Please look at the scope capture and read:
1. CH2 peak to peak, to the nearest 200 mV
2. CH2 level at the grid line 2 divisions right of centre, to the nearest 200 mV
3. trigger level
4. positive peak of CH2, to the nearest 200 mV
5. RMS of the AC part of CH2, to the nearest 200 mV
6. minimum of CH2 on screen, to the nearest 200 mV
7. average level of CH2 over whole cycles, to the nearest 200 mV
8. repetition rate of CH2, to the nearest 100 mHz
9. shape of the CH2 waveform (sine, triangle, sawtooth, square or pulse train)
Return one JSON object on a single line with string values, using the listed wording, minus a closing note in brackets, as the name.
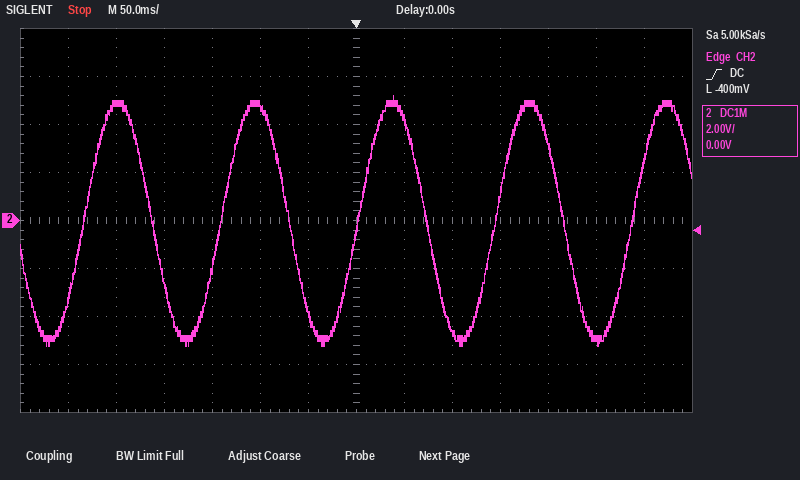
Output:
{"CH2 peak to peak, to the nearest 200 mV": "10.4 V", "CH2 level at the grid line 2 divisions right of centre, to the nearest 200 mV": "-4.6 V", "trigger level": "-400 mV", "positive peak of CH2, to the nearest 200 mV": "5.2 V", "RMS of the AC part of CH2, to the nearest 200 mV": "3.6 V", "minimum of CH2 on screen, to the nearest 200 mV": "-5.2 V", "average level of CH2 over whole cycles, to the nearest 200 mV": "0.0 V", "repetition rate of CH2, to the nearest 100 mHz": "7.0 Hz", "shape of the CH2 waveform": "sine"}
